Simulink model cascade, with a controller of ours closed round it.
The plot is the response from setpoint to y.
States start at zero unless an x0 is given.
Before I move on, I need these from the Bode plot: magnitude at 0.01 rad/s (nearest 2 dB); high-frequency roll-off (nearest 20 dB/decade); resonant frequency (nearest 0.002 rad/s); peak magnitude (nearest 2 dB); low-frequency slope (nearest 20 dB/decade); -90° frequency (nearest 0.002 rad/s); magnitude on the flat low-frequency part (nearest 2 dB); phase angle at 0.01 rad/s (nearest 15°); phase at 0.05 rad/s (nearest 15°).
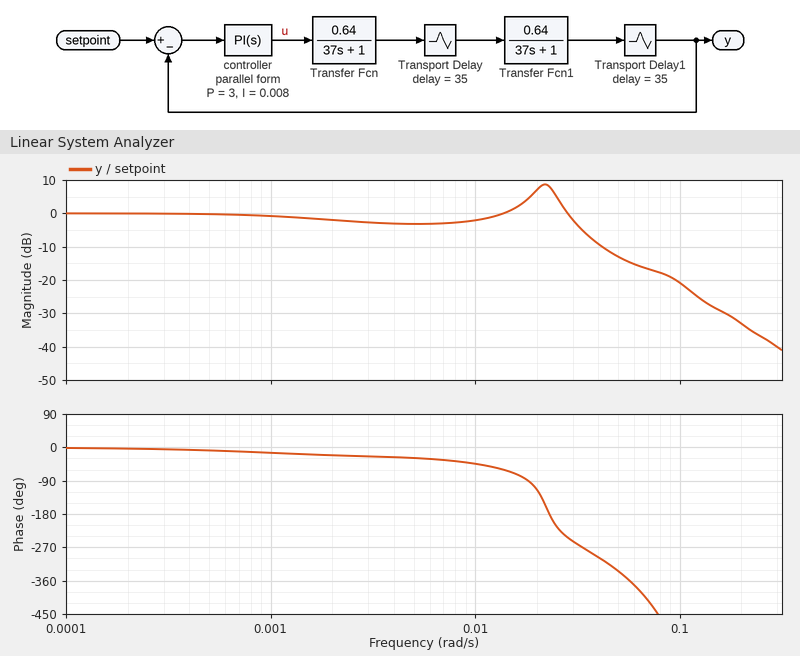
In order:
-2 dB
-40 dB/decade
0.022 rad/s
8 dB
0 dB/decade
0.018 rad/s
0 dB
-45°
-330°
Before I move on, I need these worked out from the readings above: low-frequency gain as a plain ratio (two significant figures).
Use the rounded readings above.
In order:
1.0
